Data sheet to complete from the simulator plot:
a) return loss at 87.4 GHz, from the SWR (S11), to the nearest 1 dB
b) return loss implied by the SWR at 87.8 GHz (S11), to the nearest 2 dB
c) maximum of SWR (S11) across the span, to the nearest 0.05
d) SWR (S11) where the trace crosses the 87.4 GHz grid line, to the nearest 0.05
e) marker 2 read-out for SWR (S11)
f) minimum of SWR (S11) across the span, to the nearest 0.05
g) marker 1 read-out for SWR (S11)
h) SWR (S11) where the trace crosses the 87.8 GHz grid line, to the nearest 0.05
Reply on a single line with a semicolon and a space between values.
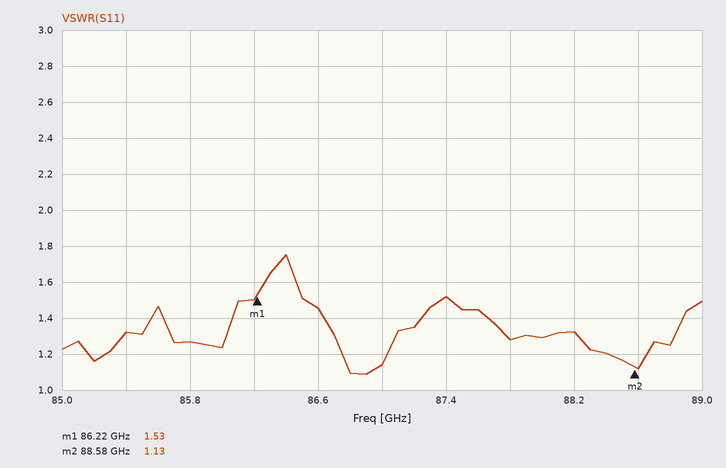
14 dB; 18 dB; 1.75; 1.50; 1.13; 1.10; 1.53; 1.30
